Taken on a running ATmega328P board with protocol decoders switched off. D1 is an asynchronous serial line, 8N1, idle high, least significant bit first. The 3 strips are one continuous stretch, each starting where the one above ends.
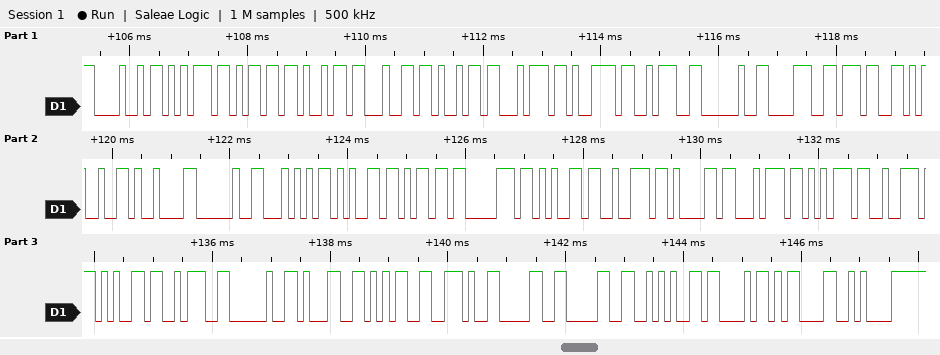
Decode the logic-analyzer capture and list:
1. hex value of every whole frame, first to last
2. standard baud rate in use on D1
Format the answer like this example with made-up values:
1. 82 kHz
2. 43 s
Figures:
1. 48 75 6D 69 64 69 74 79 3A 20 38 37 25 09 20 54 65 6D 70 65 72 61 74 75 72 65 3A 20 31 35 2E 30 30 2A 43 0D 0A
2. 9600 baud
